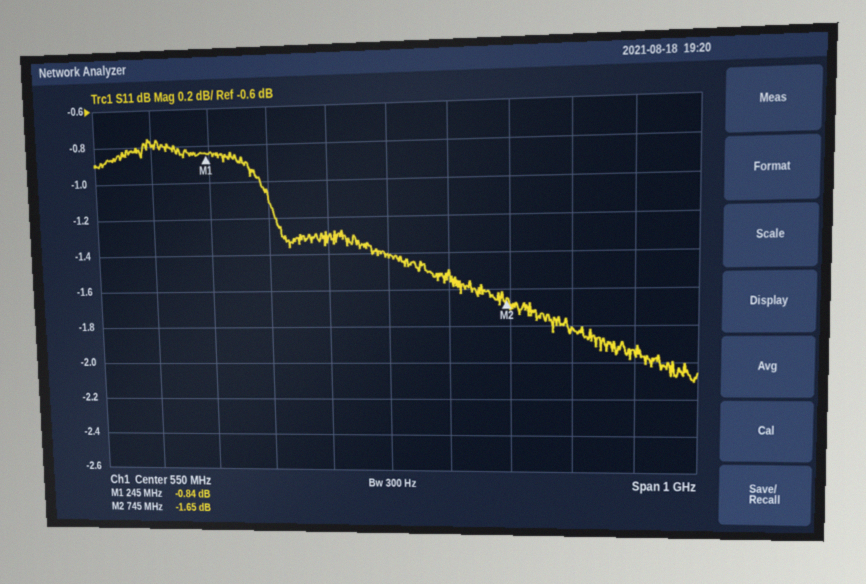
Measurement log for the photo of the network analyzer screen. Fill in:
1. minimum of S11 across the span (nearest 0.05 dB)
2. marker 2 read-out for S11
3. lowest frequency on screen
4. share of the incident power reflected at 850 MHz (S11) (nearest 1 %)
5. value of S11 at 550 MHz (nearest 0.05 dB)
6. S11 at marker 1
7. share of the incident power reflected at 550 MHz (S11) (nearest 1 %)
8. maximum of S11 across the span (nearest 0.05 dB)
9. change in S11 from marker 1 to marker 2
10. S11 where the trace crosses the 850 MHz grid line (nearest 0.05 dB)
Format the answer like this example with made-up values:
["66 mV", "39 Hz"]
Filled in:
["-2.10 dB", "-1.65 dB", "50 MHz", "66 %", "-1.40 dB", "-0.84 dB", "72 %", "-0.75 dB", "-0.81 dB", "-1.80 dB"]
